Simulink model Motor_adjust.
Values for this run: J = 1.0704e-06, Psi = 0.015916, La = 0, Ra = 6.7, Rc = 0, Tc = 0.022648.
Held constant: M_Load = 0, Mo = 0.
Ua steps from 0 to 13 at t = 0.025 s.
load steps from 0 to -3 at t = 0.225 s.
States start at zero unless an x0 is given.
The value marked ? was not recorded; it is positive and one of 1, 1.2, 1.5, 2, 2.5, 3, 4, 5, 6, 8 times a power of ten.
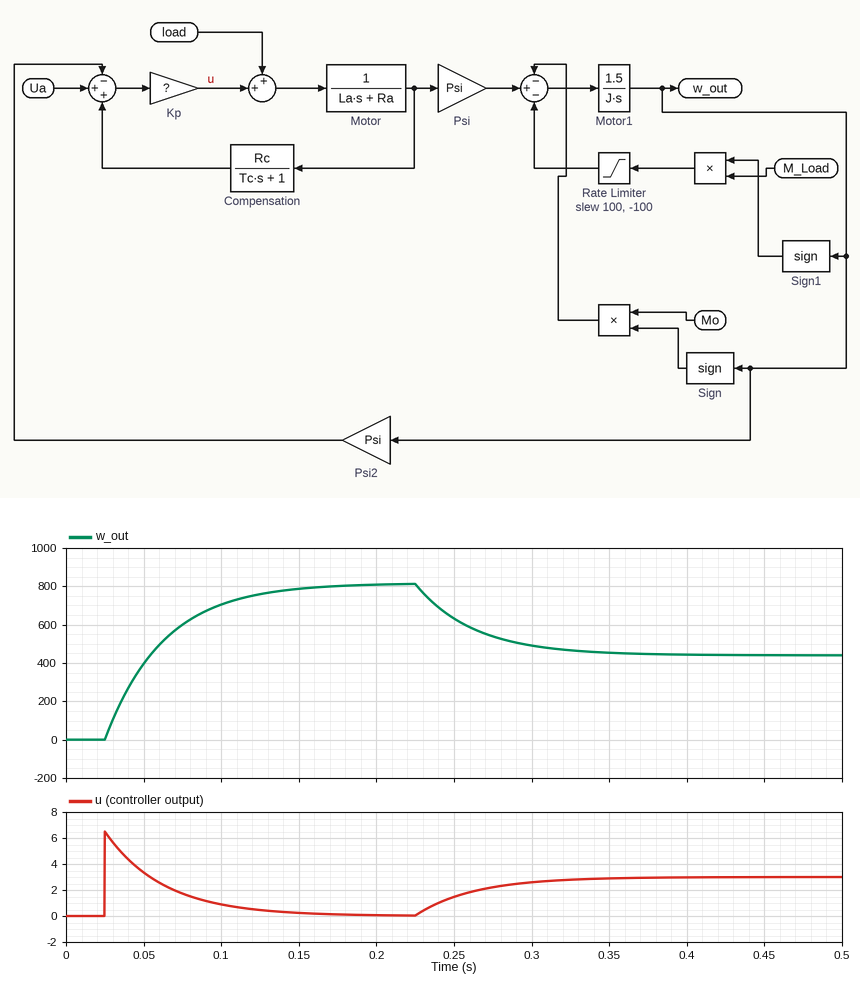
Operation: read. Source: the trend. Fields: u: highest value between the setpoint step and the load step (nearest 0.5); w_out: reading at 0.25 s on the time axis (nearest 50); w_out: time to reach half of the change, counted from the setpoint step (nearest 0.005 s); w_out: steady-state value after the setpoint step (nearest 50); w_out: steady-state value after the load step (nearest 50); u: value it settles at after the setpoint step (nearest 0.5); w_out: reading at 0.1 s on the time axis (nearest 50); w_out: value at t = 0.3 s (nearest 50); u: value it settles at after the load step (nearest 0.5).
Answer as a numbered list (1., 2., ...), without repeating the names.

1. 6.5
2. 650
3. 0.025 s
4. 800
5. 450
6. 0.0
7. 700
8. 500
9. 3.0
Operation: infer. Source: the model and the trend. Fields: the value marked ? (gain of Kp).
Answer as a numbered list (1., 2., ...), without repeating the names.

1. 0.5
